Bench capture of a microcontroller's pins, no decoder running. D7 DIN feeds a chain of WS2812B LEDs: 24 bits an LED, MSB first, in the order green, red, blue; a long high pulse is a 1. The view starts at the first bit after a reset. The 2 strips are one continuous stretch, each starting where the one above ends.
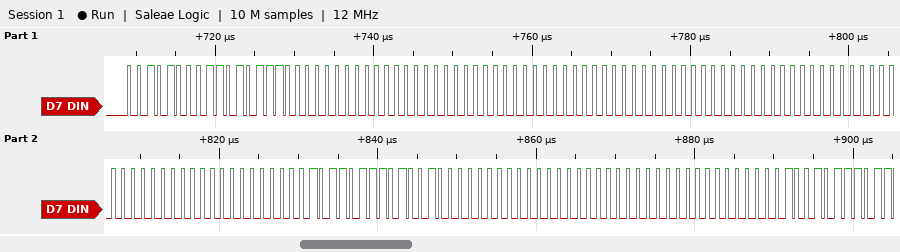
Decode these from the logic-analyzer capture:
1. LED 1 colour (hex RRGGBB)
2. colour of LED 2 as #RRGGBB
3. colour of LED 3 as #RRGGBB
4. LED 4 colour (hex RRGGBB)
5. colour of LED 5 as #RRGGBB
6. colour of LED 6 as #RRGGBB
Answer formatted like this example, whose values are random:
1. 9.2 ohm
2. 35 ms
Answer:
1. #D72800
2. #000000
3. #000000
4. #000000
5. #D22D00
6. #000000
